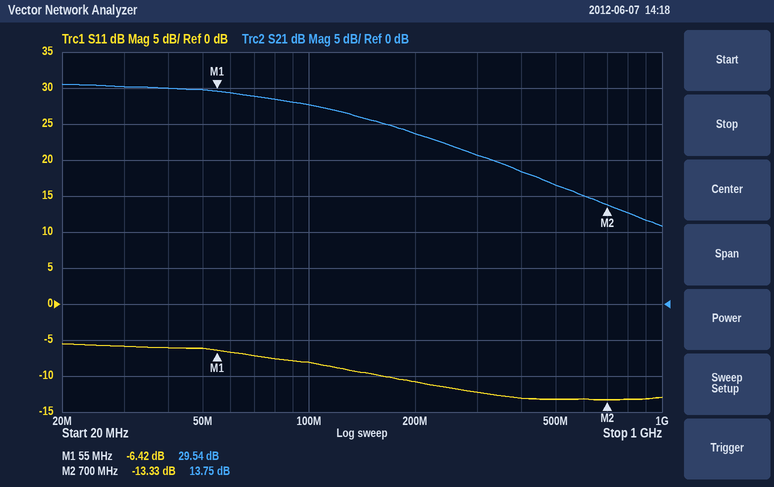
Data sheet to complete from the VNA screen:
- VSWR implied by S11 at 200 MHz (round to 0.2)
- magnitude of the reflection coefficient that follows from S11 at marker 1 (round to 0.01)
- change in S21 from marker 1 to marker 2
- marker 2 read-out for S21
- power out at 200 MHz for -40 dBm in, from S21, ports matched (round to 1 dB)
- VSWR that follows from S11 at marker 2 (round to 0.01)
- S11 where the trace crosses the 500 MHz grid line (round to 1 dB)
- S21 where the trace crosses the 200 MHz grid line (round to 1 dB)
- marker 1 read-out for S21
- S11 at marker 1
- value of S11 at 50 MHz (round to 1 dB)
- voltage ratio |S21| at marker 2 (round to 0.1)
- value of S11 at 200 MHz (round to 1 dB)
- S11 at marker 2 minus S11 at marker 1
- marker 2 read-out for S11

1.8
0.48
-15.79 dB
13.75 dB
-16 dBm
1.55
-13 dB
24 dB
29.54 dB
-6.42 dB
-6 dB
4.9
-11 dB
-6.91 dB
-13.33 dB
